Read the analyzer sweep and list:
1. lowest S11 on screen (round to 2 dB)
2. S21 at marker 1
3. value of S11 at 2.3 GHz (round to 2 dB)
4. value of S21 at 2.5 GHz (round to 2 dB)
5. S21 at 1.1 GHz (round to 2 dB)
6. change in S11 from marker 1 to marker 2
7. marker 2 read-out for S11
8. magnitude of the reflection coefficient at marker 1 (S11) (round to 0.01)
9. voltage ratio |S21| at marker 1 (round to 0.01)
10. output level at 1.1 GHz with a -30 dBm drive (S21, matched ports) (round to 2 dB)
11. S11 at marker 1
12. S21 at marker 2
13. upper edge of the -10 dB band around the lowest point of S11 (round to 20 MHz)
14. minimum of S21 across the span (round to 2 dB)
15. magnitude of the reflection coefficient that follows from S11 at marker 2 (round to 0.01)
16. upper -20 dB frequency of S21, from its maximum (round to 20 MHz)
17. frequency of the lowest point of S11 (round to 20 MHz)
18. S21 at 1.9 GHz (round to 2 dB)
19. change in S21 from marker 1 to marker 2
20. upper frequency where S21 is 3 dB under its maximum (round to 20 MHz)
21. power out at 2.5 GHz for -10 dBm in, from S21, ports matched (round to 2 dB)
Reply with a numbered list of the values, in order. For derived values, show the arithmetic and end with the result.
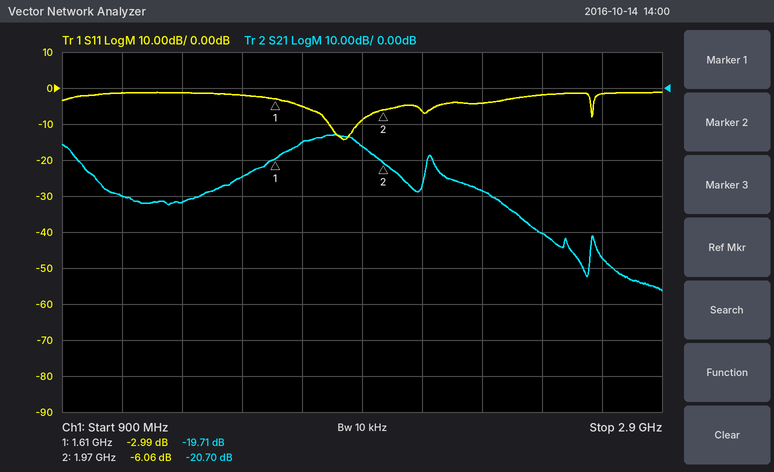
1. -14 dB
2. -19.71 dB
3. -4 dB
4. -40 dB
5. -30 dB
6. -6.06 − (-2.99) = -3.07 dB
7. -6.06 dB
8. 10^(-2.99/20) ≈ 0.71
9. 10^(-19.71/20) ≈ 0.10
10. -30 dBm + (-30 dB) = -60 dBm
11. -2.99 dB
12. -20.70 dB
13. 1.88 GHz
14. -56 dB
15. 10^(-6.06/20) ≈ 0.50
16. 2.38 GHz
17. 1.84 GHz
18. -16 dB
19. -20.7 − (-19.71) = -0.99 dB
20. 1.90 GHz
21. -10 dBm + (-40 dB) = -50 dBm
